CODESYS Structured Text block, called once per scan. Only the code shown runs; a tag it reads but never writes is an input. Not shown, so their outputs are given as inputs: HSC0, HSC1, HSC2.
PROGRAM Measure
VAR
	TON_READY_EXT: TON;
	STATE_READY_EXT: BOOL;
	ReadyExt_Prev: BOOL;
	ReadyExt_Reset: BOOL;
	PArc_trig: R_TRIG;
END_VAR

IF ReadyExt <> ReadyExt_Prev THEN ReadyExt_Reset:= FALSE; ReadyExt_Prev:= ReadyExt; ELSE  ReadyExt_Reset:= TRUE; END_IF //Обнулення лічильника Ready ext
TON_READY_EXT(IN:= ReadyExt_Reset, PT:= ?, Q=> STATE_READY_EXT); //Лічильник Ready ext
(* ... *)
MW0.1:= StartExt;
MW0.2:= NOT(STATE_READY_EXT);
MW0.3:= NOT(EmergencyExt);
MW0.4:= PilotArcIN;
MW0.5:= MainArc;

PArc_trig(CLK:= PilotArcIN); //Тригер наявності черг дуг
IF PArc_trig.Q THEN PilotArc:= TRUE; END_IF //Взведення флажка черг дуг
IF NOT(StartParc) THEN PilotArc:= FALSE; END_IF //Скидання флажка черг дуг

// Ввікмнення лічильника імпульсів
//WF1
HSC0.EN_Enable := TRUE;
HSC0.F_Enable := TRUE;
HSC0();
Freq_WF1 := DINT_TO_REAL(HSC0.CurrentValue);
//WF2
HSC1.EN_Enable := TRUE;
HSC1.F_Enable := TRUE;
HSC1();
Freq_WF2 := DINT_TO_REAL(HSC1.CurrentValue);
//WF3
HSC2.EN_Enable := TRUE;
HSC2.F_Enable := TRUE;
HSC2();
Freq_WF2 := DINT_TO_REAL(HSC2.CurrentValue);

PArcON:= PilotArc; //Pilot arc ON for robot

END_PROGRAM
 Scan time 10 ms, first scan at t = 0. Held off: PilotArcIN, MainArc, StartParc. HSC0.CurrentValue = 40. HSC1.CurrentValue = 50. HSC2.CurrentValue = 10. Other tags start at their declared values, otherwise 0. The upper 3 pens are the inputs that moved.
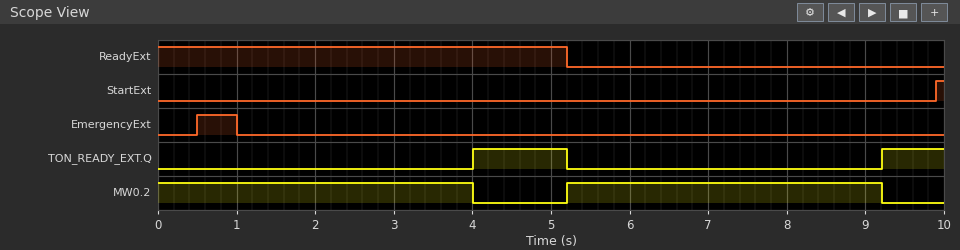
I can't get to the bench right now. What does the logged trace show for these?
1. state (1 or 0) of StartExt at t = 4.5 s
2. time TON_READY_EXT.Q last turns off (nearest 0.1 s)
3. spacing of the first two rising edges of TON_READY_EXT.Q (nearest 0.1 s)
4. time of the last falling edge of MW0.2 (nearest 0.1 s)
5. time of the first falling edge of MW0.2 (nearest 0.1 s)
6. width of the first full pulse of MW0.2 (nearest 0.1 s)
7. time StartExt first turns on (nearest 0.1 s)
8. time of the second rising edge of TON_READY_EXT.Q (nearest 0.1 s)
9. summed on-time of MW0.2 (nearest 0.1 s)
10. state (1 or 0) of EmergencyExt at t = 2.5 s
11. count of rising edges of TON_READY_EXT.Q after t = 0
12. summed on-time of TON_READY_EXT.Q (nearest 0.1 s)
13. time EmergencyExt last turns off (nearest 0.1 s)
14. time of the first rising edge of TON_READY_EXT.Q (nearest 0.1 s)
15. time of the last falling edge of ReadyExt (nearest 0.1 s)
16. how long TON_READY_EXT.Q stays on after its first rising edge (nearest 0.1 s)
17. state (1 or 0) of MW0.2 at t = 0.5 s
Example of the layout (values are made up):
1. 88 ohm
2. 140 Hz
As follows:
1. 0
2. 5.2 s
3. 5.2 s
4. 9.2 s
5. 4.0 s
6. 4.0 s
7. 9.9 s
8. 9.2 s
9. 8.0 s
10. 0
11. 2
12. 2.0 s
13. 1.0 s
14. 4.0 s
15. 5.2 s
16. 1.2 s
17. 1
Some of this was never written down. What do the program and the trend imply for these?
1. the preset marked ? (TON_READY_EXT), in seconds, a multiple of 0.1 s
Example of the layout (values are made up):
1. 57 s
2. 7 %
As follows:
1. 4.0 s
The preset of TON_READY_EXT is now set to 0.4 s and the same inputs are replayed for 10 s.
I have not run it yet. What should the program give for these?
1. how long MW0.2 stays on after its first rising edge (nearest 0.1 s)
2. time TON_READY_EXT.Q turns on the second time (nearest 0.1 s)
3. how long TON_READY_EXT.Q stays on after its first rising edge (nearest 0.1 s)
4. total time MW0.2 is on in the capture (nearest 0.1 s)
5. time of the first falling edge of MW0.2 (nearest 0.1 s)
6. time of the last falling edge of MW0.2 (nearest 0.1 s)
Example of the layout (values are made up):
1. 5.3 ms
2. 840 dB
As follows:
1. 0.4 s
2. 5.6 s
3. 4.8 s
4. 0.8 s
5. 0.4 s
6. 5.6 s
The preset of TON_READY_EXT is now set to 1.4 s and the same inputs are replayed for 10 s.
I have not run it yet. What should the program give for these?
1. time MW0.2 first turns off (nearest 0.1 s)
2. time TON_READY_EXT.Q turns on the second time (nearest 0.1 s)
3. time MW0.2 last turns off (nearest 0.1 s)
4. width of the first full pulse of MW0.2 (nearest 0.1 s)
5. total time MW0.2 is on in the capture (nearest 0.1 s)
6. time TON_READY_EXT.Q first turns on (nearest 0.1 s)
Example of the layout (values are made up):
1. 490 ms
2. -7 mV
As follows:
1. 1.4 s
2. 6.6 s
3. 6.6 s
4. 1.4 s
5. 2.8 s
6. 1.4 s
